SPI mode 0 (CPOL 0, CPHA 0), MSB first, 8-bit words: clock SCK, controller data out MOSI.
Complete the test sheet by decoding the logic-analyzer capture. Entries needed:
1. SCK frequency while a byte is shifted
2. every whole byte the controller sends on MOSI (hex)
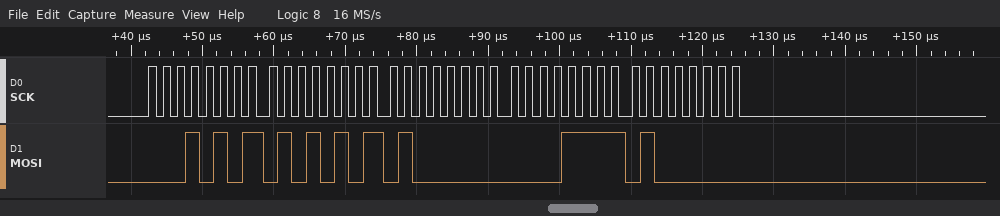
500 kHz
0x15 0x55 0x40 0x0F 0x40
